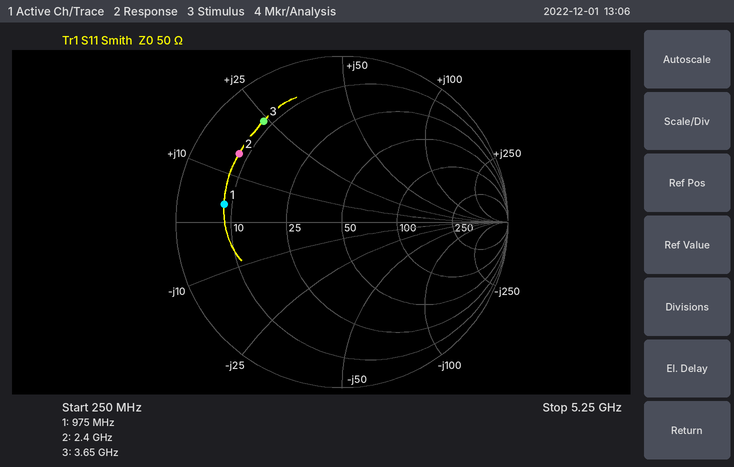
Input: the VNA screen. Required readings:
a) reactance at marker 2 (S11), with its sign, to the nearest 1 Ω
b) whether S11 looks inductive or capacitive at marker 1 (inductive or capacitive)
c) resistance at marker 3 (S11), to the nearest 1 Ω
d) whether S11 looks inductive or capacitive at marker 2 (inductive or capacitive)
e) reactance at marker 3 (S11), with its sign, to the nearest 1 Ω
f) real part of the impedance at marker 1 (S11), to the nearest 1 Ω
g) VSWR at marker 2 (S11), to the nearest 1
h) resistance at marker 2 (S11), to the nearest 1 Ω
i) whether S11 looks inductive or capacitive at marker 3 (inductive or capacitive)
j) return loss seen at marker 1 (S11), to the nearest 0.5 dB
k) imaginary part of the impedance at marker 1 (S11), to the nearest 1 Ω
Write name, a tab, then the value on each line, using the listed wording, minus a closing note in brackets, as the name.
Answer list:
reactance at marker 2 (S11), with its sign, to the nearest 1 Ω	+15 Ω
whether S11 looks inductive or capacitive at marker 1	inductive
resistance at marker 3 (S11), to the nearest 1 Ω	8 Ω
whether S11 looks inductive or capacitive at marker 2	inductive
reactance at marker 3 (S11), with its sign, to the nearest 1 Ω	+24 Ω
real part of the impedance at marker 1 (S11), to the nearest 1 Ω	8 Ω
VSWR at marker 2 (S11), to the nearest 1	7
resistance at marker 2 (S11), to the nearest 1 Ω	8 Ω
whether S11 looks inductive or capacitive at marker 3	inductive
return loss seen at marker 1 (S11), to the nearest 0.5 dB	3.0 dB
imaginary part of the impedance at marker 1 (S11), to the nearest 1 Ω	+4 Ω
